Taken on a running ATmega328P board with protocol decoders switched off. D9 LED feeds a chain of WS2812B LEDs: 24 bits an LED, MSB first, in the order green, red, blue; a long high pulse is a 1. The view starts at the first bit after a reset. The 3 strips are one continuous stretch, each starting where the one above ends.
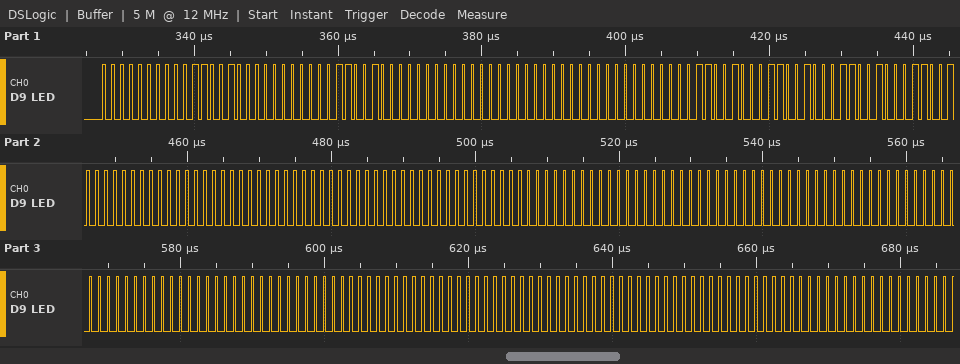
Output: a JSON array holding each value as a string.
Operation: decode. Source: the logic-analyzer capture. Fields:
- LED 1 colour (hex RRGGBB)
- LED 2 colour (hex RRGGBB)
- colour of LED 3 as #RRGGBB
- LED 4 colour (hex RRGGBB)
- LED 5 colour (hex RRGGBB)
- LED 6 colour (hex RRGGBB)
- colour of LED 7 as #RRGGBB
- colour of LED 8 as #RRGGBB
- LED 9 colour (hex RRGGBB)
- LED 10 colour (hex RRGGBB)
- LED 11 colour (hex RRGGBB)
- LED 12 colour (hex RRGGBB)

["#320000", "#003200", "#000032", "#323232", "#000000", "#000000", "#000000", "#000000", "#000000", "#000000", "#000000", "#000000"]
